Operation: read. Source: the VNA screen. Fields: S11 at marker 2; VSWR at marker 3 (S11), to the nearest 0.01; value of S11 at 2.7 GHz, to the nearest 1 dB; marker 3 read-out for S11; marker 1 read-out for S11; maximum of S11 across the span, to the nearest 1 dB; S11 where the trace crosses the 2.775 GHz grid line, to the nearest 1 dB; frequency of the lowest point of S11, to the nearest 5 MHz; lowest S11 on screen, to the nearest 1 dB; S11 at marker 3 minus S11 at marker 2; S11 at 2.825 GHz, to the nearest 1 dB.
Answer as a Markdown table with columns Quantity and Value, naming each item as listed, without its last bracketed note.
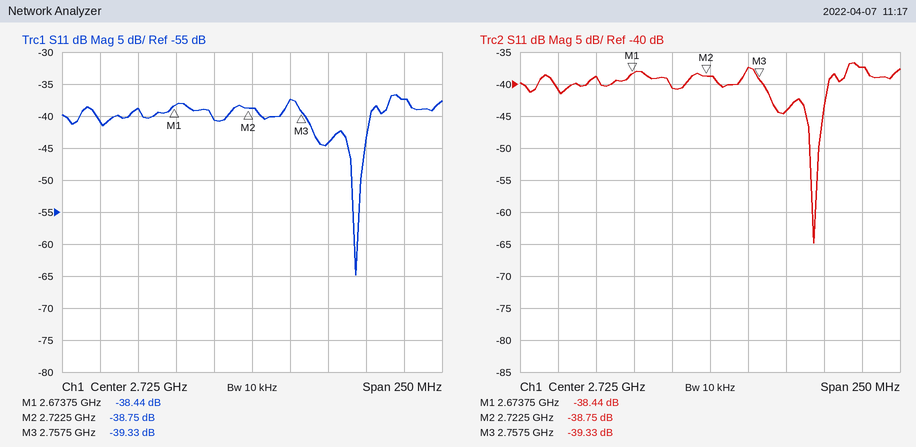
| Quantity | Value |
|---|---|
| S11 at marker 2 | -38.75 dB |
| VSWR at marker 3 (S11), to the nearest 0.01 | 1.02 |
| value of S11 at 2.7 GHz, to the nearest 1 dB | -41 dB |
| marker 3 read-out for S11 | -39.33 dB |
| marker 1 read-out for S11 | -38.44 dB |
| maximum of S11 across the span, to the nearest 1 dB | -37 dB |
| S11 where the trace crosses the 2.775 GHz grid line, to the nearest 1 dB | -44 dB |
| frequency of the lowest point of S11, to the nearest 5 MHz | 2.795 GHz |
| lowest S11 on screen, to the nearest 1 dB | -65 dB |
| S11 at marker 3 minus S11 at marker 2 | -0.58 dB |
| S11 at 2.825 GHz, to the nearest 1 dB | -37 dB |
